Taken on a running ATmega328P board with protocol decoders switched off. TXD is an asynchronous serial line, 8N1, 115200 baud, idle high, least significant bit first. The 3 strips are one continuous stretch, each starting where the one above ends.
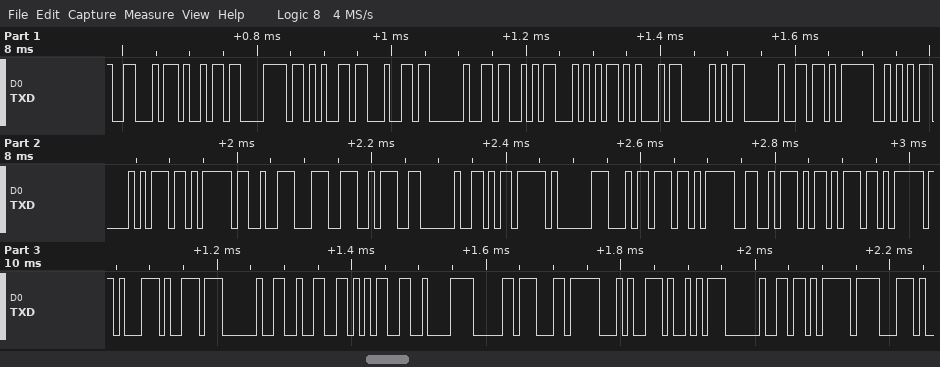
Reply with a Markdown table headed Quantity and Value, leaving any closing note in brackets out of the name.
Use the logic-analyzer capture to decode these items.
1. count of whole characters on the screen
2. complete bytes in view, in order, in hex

| Quantity | Value |
|---|---|
| count of whole characters on the screen | 39 |
| complete bytes in view, in order, in hex | 46 69 78 65 64 20 53 54 45 50 20 EB AA A8 EB 93 9C 3A 20 ED 81 B4 EB A6 AD EB 8B B9 20 32 35 C2 B0 EC 94 A9 20 EB 8F |
